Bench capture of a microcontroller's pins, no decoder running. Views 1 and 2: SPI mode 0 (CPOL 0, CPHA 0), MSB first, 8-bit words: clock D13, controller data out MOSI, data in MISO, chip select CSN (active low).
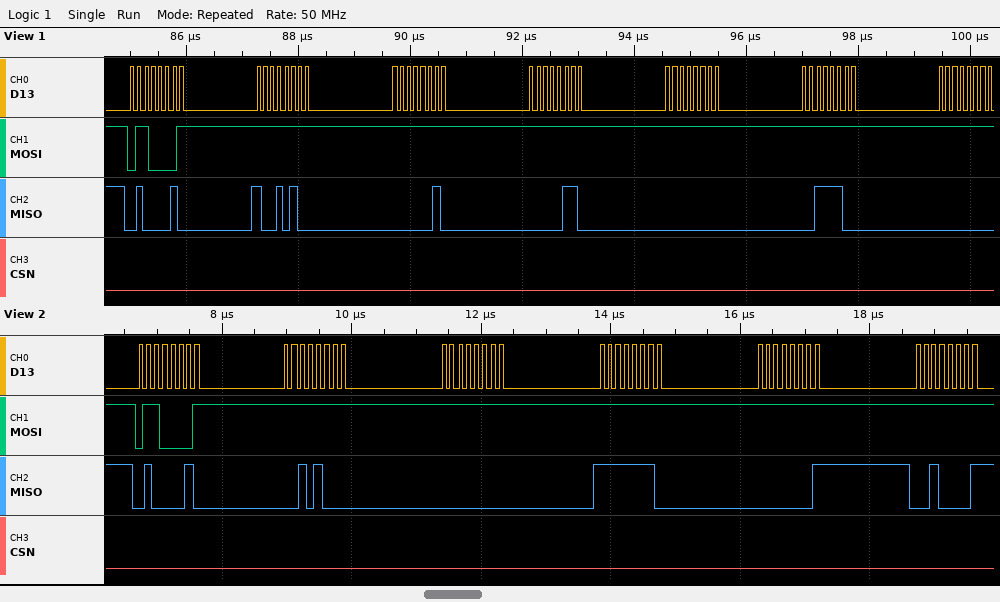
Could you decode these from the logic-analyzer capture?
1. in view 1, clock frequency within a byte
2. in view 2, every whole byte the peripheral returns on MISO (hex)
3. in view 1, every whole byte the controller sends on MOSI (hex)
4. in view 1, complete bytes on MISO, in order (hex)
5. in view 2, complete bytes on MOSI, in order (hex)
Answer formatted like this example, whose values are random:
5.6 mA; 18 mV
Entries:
8 MHz; 42 28 00 FE 01 21; 61 FF FF FF FF FF FF; 42 94 02 06 00 3C 00; 61 FF FF FF FF FF
